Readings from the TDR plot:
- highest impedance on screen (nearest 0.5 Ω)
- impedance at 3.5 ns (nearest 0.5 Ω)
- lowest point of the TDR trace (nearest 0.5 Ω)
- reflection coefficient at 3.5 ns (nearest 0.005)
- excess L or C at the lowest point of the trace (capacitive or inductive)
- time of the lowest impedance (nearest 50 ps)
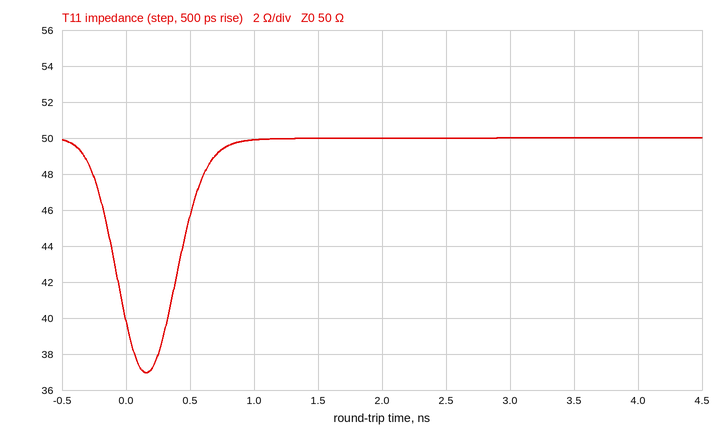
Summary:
50.0 Ω
50.0 Ω
37.0 Ω
0.000
capacitive
150 ps
